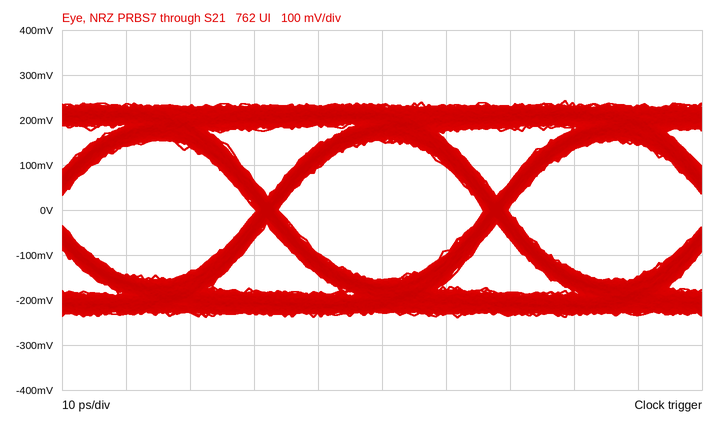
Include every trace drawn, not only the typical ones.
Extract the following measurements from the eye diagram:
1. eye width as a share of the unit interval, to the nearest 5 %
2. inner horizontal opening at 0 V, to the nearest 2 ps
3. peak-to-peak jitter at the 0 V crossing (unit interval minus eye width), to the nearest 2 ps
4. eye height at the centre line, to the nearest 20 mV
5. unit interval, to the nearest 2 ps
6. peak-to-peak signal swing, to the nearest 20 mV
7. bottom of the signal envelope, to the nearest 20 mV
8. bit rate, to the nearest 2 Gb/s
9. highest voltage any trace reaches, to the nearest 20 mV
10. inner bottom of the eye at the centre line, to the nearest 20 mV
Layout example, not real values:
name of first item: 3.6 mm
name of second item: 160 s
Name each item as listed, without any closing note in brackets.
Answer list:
eye width as a share of the unit interval, to the nearest 5 %: 90 %
inner horizontal opening at 0 V, to the nearest 2 ps: 32 ps
peak-to-peak jitter at the 0 V crossing (unit interval minus eye width), to the nearest 2 ps: 4 ps
eye height at the centre line, to the nearest 20 mV: 300 mV
unit interval, to the nearest 2 ps: 36 ps
peak-to-peak signal swing, to the nearest 20 mV: 480 mV
bottom of the signal envelope, to the nearest 20 mV: -240 mV
bit rate, to the nearest 2 Gb/s: 28 Gb/s
highest voltage any trace reaches, to the nearest 20 mV: 240 mV
inner bottom of the eye at the centre line, to the nearest 20 mV: -160 mV
